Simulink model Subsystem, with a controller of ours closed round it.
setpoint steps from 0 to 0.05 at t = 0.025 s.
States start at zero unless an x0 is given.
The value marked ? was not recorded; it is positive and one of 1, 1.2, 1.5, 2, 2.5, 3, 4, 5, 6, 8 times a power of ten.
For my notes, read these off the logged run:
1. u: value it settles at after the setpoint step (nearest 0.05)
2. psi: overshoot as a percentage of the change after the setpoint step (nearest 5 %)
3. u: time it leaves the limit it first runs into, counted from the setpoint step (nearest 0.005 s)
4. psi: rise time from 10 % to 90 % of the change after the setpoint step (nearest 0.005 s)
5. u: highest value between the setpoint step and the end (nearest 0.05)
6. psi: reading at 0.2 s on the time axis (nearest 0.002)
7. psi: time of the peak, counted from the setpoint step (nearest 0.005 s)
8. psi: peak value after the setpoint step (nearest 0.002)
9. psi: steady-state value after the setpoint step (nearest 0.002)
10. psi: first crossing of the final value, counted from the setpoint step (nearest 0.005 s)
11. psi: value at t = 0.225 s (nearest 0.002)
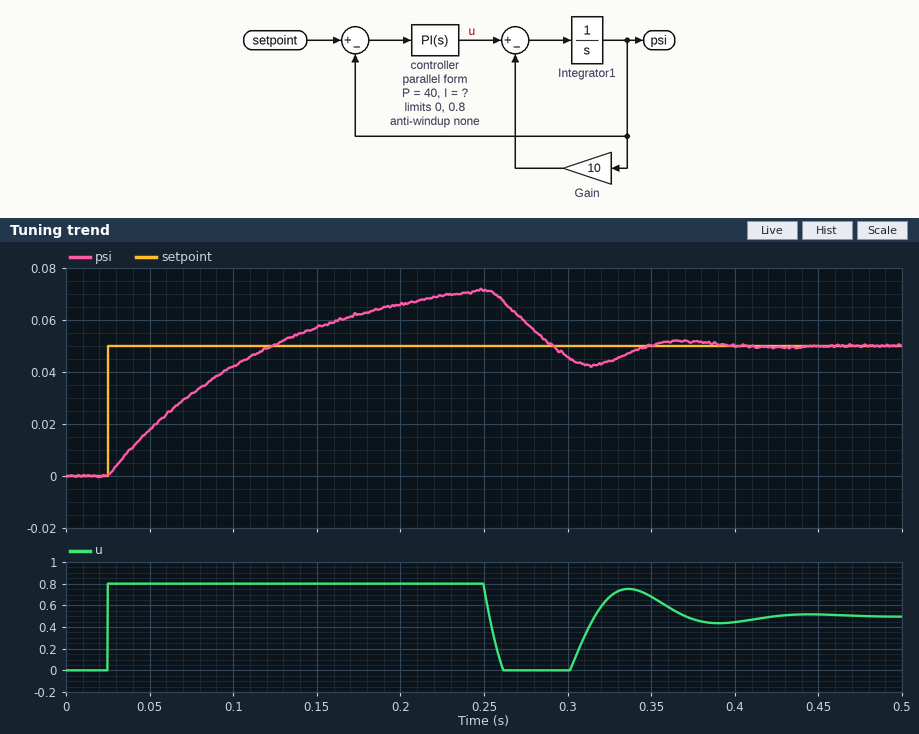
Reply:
0.50
45 %
0.225 s
0.075 s
0.80
0.066
0.225 s
0.072
0.050
0.100 s
0.070
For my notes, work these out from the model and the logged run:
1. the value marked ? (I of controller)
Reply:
4000
